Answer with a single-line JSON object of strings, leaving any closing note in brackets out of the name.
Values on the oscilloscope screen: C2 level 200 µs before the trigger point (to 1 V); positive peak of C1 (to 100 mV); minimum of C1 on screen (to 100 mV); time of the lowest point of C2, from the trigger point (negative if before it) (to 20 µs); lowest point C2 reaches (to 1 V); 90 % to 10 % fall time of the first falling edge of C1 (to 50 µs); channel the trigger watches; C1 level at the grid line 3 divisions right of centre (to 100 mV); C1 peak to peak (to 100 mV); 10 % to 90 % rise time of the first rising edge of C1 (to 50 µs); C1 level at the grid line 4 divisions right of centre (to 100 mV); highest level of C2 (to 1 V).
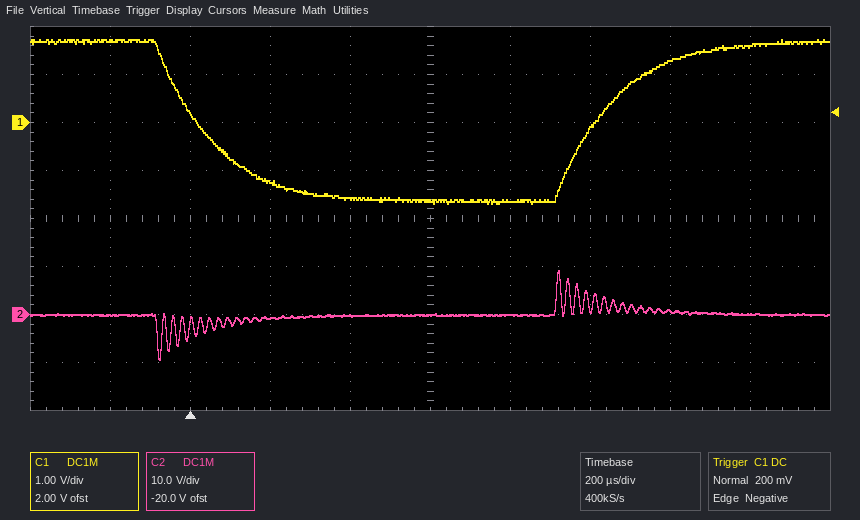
{"C2 level 200 µs before the trigger point": "0 V", "positive peak of C1": "1.7 V", "minimum of C1 on screen": "-1.7 V", "time of the lowest point of C2, from the trigger point (negative if before it)": "-80 µs", "lowest point C2 reaches": "-9 V", "90 % to 10 % fall time of the first falling edge of C1": "300 µs", "channel the trigger watches": "C1", "C1 level at the grid line 3 divisions right of centre": "1.3 V", "C1 peak to peak": "3.4 V", "10 % to 90 % rise time of the first rising edge of C1": "300 µs", "C1 level at the grid line 4 divisions right of centre": "1.6 V", "highest level of C2": "9 V"}
